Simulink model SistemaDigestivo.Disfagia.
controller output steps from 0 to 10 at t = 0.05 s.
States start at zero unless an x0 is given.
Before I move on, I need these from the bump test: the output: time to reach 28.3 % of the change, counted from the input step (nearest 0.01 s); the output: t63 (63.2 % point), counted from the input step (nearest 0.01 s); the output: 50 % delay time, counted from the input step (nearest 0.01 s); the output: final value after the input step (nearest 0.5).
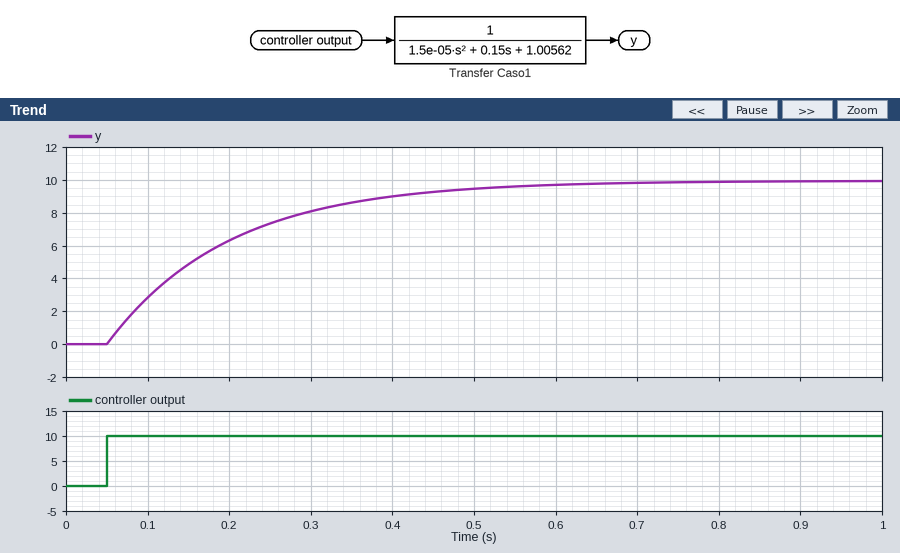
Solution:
0.05 s
0.15 s
0.10 s
10.0
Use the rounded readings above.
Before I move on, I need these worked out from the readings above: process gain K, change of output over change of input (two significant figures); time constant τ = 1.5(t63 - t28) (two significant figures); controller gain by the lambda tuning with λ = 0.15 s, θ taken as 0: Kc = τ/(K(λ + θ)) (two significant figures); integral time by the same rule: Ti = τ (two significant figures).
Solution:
1.0
0.15 s
1.0
0.15 s
